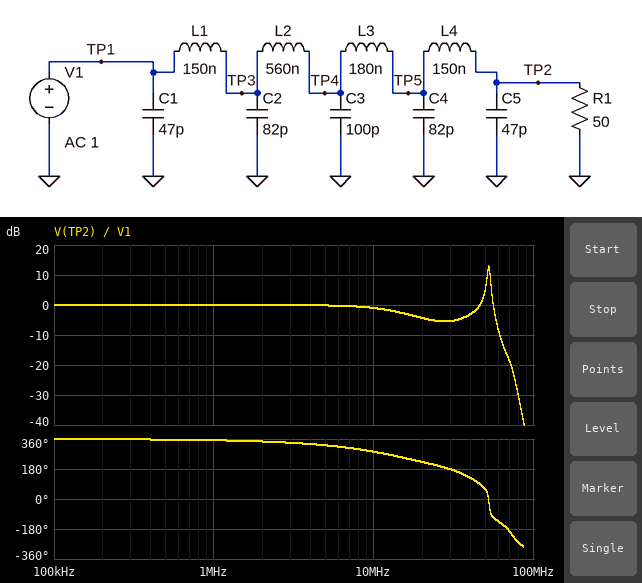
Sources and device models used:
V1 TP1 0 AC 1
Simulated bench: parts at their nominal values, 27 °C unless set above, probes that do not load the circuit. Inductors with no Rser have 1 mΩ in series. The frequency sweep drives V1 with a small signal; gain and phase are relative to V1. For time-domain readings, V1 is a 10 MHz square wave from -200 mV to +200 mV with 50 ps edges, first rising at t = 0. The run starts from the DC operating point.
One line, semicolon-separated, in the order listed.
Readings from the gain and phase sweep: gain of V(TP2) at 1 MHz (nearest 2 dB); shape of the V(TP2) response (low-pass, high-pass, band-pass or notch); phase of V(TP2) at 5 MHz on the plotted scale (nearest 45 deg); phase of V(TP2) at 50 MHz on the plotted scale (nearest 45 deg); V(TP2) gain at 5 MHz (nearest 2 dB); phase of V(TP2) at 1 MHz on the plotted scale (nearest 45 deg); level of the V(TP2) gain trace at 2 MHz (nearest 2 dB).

0 dB; band-pass; 315 deg; 45 deg; 0 dB; 360 deg; 0 dB
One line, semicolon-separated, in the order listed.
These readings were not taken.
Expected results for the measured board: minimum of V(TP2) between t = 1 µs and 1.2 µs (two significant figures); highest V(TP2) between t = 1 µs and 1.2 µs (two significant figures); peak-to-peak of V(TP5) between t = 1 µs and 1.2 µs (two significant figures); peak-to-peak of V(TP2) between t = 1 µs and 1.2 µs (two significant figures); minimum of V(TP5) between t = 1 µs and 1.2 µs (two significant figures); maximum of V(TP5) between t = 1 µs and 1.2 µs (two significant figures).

-280 mV; 280 mV; 560 mV; 560 mV; -280 mV; 280 mV
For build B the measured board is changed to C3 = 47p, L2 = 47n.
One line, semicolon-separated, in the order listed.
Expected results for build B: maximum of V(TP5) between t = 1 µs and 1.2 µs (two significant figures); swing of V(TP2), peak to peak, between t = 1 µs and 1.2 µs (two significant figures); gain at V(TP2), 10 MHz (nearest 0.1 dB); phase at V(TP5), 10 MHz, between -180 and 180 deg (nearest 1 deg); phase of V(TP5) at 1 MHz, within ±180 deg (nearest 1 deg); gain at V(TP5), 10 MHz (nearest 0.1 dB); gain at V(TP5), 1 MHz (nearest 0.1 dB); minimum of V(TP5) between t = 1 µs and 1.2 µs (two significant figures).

300 mV; 630 mV; 0.6 dB; -29 deg; -3 deg; 0.5 dB; 0 dB; -300 mV
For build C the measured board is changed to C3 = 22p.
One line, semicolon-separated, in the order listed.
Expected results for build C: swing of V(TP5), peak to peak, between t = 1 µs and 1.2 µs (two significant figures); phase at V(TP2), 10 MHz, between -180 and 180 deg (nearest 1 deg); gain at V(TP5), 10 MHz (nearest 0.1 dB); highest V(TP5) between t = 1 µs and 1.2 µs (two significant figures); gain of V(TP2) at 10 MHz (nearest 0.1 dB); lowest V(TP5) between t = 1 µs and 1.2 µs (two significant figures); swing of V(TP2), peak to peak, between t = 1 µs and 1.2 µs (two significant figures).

720 mV; -69 deg; -2.1 dB; 360 mV; -2.0 dB; -360 mV; 740 mV
